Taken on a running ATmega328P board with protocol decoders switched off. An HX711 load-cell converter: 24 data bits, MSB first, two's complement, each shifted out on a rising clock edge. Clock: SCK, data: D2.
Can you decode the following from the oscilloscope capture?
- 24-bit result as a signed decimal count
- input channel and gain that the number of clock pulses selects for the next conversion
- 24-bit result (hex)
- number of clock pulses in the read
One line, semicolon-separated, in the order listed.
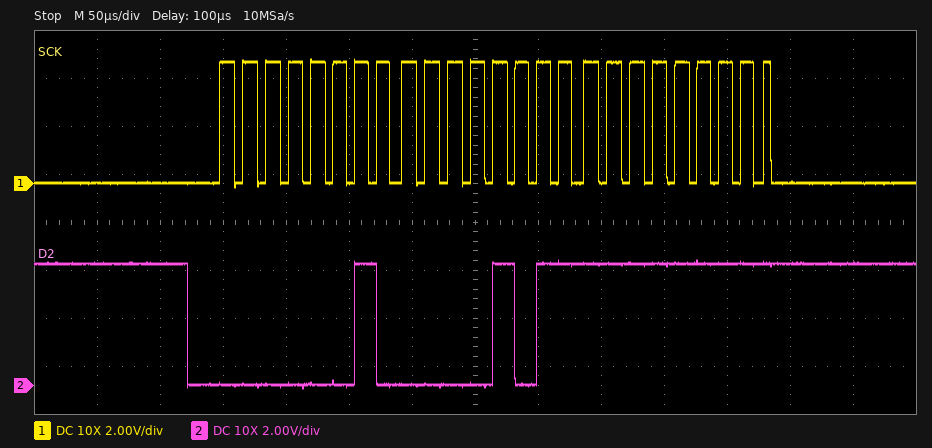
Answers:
134143; channel A, gain 128; 0x020BFF; 25
